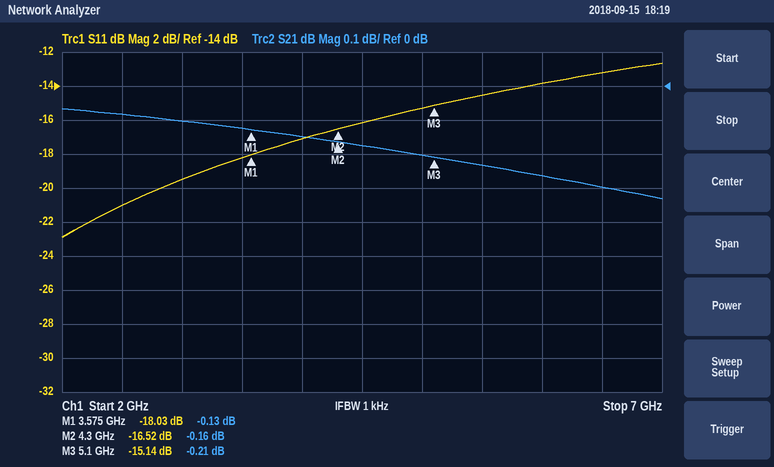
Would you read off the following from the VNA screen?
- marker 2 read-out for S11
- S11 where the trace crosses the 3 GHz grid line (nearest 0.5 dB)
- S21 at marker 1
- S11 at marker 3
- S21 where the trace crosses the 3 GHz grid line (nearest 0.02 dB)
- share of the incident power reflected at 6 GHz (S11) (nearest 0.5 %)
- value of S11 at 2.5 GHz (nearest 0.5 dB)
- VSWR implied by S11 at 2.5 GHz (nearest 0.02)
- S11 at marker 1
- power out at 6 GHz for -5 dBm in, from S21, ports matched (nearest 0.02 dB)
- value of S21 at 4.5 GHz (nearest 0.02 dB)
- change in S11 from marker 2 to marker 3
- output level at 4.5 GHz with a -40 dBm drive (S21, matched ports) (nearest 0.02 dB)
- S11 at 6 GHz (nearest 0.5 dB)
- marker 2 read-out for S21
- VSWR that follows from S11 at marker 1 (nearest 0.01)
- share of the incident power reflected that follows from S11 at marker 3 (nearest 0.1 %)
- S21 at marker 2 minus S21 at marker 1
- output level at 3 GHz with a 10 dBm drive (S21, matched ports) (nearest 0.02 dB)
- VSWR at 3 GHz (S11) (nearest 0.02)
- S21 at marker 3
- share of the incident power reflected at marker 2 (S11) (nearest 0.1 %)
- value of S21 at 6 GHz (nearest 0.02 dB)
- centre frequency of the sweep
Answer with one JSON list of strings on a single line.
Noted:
["-16.52 dB", "-19.5 dB", "-0.13 dB", "-15.14 dB", "-0.10 dB", "4.0 %", "-21.0 dB", "1.20", "-18.03 dB", "-5.26 dBm", "-0.18 dB", "1.38 dB", "-40.18 dBm", "-14.0 dB", "-0.16 dB", "1.29", "3.1 %", "-0.03 dB", "9.90 dBm", "1.24", "-0.21 dB", "2.2 %", "-0.26 dB", "4.5 GHz"]
